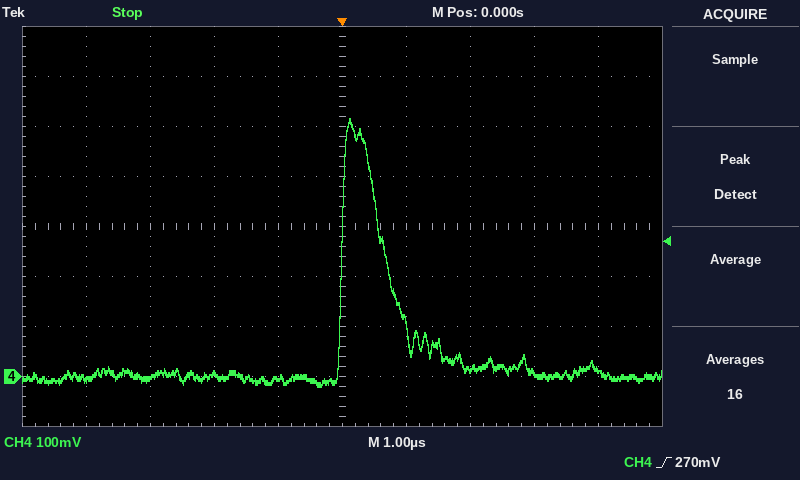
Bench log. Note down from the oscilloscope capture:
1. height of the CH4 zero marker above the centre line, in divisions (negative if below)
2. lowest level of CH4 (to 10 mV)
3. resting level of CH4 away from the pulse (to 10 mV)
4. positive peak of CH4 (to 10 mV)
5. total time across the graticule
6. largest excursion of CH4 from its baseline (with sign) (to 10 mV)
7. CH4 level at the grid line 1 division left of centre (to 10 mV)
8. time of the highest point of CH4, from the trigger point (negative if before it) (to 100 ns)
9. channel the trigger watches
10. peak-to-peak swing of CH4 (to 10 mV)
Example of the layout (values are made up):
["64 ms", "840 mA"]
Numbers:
["-3.0 div", "-20 mV", "0 mV", "520 mV", "10 µs", "+520 mV", "0 mV", "+100 ns", "CH4", "540 mV"]
